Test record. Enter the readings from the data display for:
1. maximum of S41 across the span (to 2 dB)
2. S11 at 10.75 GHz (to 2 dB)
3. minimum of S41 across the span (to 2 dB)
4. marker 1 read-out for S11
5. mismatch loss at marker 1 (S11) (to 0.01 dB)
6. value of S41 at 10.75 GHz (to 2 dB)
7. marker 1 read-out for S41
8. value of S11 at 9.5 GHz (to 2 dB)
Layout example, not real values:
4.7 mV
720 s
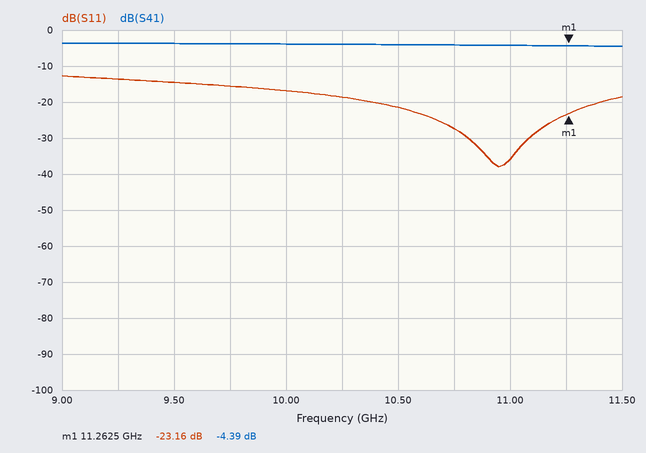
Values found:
-4 dB
-28 dB
-4 dB
-23.16 dB
0.02 dB
-4 dB
-4.39 dB
-14 dB
